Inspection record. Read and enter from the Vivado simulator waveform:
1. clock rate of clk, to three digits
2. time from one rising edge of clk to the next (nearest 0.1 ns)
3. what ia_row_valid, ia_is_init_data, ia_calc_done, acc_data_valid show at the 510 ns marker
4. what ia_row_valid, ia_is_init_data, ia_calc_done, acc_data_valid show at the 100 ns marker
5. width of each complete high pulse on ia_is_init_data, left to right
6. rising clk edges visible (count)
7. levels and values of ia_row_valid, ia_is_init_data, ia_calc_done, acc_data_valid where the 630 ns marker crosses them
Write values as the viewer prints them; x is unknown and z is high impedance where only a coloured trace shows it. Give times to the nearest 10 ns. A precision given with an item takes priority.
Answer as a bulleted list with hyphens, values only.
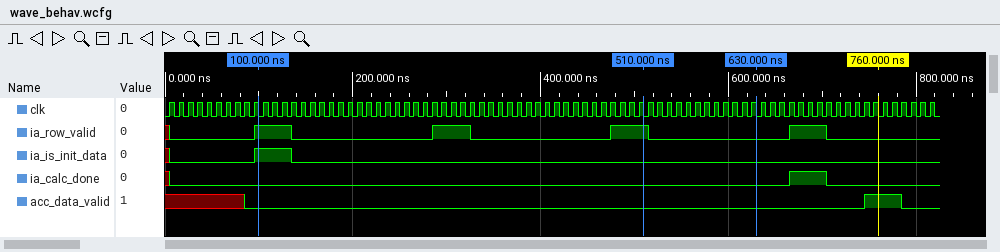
- 100 MHz
- 10 ns
- ia_row_valid=1, ia_is_init_data=0, ia_calc_done=0, acc_data_valid=0
- ia_row_valid=1, ia_is_init_data=1, ia_calc_done=0, acc_data_valid=0
- 40 ns
- 82
- ia_row_valid=0, ia_is_init_data=0, ia_calc_done=0, acc_data_valid=0
